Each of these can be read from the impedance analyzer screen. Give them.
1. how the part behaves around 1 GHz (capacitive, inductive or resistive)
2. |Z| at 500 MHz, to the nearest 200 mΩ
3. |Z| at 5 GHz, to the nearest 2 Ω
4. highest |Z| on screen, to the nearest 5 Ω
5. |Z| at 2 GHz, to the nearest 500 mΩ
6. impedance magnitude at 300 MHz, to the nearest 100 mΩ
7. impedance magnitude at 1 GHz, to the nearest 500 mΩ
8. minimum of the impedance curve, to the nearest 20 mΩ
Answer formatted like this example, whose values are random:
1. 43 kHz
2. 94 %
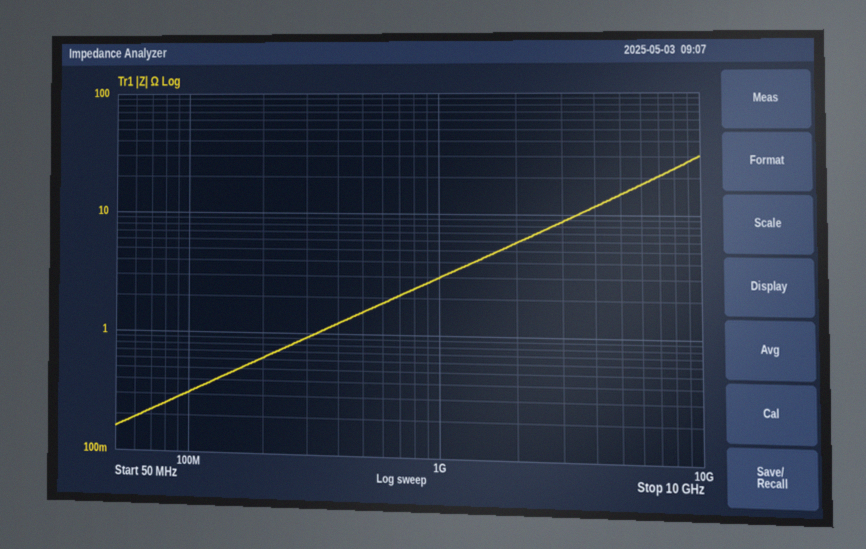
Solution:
1. inductive
2. 1.6 Ω
3. 14 Ω
4. 30 Ω
5. 6.0 Ω
6. 900 mΩ
7. 3.0 Ω
8. 160 mΩ
